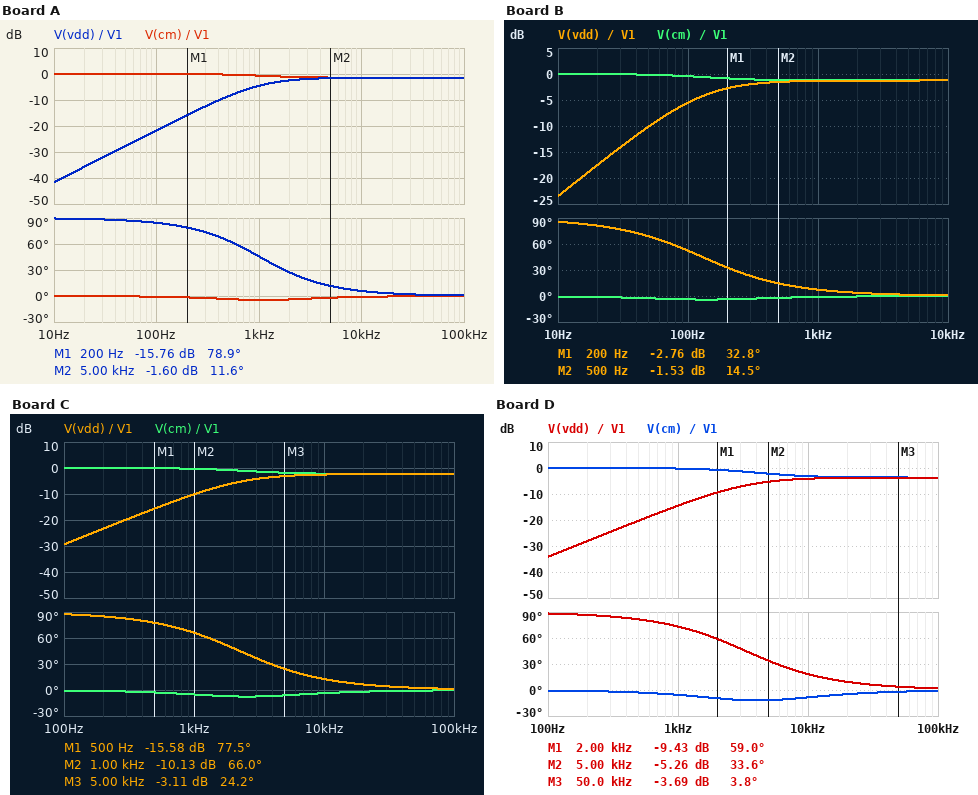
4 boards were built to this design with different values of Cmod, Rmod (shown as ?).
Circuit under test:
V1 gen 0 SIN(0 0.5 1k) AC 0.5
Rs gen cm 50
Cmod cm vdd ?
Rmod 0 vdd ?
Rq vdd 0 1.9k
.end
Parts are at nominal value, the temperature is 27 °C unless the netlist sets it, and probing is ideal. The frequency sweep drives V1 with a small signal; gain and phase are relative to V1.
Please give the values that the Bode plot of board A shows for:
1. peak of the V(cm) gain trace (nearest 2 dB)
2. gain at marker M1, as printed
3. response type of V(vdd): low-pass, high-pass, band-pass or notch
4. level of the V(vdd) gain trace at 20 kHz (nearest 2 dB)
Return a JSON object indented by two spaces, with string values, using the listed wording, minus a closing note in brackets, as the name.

{
  "peak of the V(cm) gain trace": "0 dB",
  "gain at marker M1, as printed": "-15.76 dB",
  "response type of V(vdd): low-pass, high-pass, band-pass or notch": "high-pass",
  "level of the V(vdd) gain trace at 20 kHz": "-2 dB"
}
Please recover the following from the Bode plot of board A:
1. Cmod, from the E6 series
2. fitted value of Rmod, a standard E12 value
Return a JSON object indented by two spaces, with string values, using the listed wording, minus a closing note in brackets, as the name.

{
  "Cmod, from the E6 series": "470 nF",
  "fitted value of Rmod, a standard E12 value": "330 Ω"
}
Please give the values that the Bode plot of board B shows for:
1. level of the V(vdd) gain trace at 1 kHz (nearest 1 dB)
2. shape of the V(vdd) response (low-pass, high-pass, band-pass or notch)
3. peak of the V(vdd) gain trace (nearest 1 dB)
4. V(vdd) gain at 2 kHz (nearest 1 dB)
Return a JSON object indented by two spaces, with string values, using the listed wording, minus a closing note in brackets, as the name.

{
  "level of the V(vdd) gain trace at 1 kHz": "-1 dB",
  "shape of the V(vdd) response": "high-pass",
  "peak of the V(vdd) gain trace": "-1 dB",
  "V(vdd) gain at 2 kHz": "-1 dB"
}
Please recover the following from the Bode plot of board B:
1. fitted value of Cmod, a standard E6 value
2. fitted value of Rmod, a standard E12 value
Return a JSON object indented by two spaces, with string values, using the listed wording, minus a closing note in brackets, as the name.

{
  "fitted value of Cmod, a standard E6 value": "3.3 µF",
  "fitted value of Rmod, a standard E12 value": "390 Ω"
}
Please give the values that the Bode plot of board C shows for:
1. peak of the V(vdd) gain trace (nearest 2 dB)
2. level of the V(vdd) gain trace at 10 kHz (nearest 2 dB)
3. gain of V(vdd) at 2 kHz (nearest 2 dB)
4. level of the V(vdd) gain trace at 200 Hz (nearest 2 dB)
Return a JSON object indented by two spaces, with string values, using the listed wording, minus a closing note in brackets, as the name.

{
  "peak of the V(vdd) gain trace": "-2 dB",
  "level of the V(vdd) gain trace at 10 kHz": "-2 dB",
  "gain of V(vdd) at 2 kHz": "-6 dB",
  "level of the V(vdd) gain trace at 200 Hz": "-24 dB"
}
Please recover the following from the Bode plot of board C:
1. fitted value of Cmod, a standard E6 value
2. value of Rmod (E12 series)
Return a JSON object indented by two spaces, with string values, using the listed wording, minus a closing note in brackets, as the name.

{
  "fitted value of Cmod, a standard E6 value": "330 nF",
  "value of Rmod": "180 Ω"
}
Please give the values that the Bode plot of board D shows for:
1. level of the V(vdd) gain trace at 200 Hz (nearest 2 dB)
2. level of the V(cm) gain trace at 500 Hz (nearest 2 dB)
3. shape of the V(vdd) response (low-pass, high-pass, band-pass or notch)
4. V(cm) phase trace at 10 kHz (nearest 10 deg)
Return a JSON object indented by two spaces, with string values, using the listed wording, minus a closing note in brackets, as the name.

{
  "level of the V(vdd) gain trace at 200 Hz": "-28 dB",
  "level of the V(cm) gain trace at 500 Hz": "0 dB",
  "shape of the V(vdd) response": "high-pass",
  "V(cm) phase trace at 10 kHz": "-10 deg"
}
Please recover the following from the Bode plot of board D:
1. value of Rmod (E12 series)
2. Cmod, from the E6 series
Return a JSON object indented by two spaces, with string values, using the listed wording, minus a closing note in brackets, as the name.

{
  "value of Rmod": "100 Ω",
  "Cmod, from the E6 series": "330 nF"
}
